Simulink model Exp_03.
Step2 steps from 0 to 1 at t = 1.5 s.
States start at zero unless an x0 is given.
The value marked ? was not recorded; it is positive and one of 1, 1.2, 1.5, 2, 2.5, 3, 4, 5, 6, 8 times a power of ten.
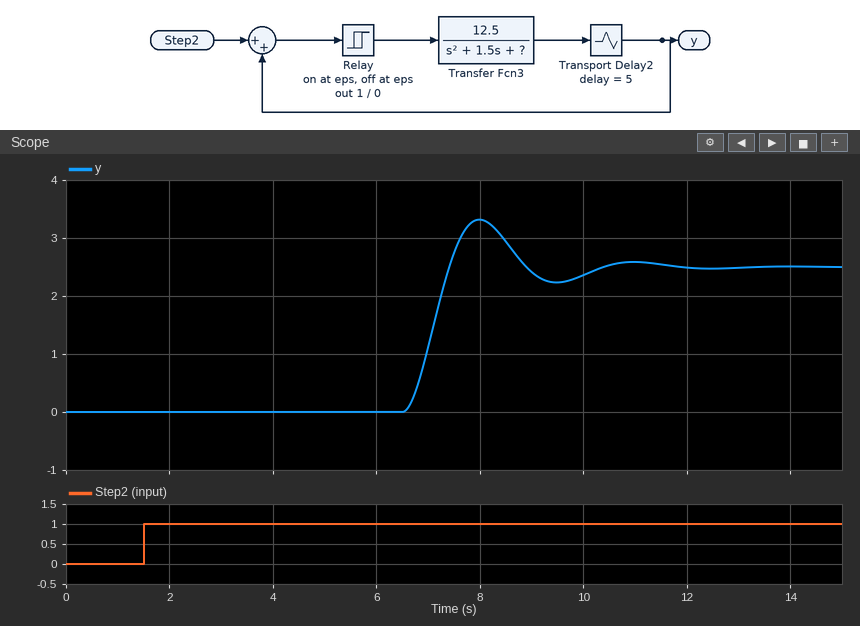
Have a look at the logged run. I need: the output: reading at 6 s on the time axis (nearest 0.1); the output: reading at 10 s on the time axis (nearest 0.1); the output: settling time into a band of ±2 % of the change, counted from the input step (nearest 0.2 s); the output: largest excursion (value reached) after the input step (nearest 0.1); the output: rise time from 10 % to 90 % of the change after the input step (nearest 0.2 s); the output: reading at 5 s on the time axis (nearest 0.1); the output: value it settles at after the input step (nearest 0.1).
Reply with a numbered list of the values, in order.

1. 0.0
2. 2.4
3. 10.0 s
4. 3.3
5. 0.6 s
6. 0.0
7. 2.5
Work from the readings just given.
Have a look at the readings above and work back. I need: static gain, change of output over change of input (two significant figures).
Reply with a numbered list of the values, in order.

1. 2.5
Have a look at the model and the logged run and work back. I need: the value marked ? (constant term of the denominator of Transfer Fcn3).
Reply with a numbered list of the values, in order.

1. 5
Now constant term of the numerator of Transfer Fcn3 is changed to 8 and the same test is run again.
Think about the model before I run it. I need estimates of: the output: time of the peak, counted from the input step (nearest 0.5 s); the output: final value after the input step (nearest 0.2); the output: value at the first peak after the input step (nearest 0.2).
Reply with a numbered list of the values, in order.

1. 6.5 s
2. 1.6
3. 2.2
